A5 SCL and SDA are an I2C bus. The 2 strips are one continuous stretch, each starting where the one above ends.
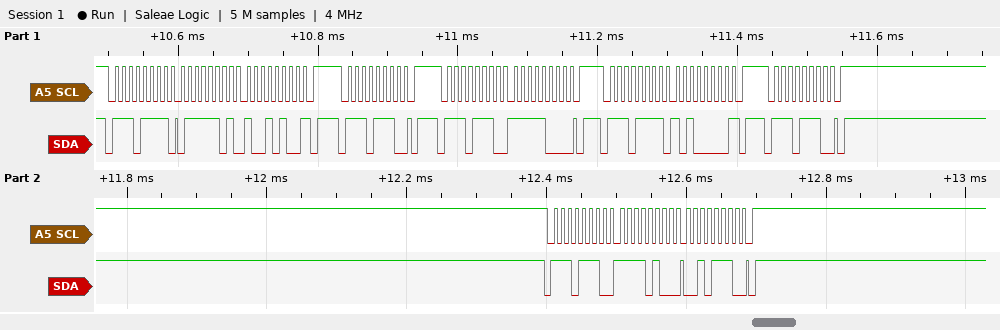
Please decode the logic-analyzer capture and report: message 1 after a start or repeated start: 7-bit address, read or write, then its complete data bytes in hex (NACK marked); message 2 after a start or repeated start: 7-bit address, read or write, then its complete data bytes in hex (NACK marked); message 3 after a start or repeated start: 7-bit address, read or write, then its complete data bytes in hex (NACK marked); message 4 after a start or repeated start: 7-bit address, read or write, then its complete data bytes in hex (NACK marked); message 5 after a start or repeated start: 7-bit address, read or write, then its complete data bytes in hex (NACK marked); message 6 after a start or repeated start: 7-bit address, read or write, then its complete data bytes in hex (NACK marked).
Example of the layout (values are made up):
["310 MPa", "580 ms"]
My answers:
["0x77 read: 7D 94 NACK", "0x77 write", "0x77 write: F8", "0x77 read: A0 NACK", "0x77 write", "0x77 write: F4 2E"]
